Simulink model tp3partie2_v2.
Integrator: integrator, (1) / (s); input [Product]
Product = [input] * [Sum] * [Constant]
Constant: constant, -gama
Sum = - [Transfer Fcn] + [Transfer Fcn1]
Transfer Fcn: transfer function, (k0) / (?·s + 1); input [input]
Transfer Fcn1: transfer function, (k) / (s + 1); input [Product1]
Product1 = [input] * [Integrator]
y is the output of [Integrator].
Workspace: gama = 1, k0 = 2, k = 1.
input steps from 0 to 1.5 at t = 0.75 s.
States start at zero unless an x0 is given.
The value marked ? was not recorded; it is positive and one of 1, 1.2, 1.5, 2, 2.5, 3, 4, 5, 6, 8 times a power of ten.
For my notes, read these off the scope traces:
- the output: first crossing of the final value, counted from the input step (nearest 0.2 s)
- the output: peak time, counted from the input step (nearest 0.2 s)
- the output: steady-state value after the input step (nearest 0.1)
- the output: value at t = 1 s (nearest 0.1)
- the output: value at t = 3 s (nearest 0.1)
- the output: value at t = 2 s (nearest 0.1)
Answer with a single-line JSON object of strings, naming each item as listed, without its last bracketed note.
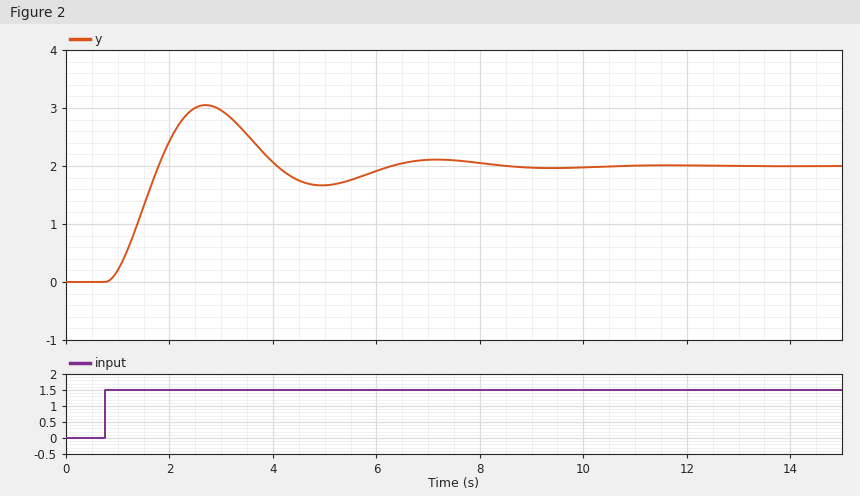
{"the output: first crossing of the final value, counted from the input step": "1.0 s", "the output: peak time, counted from the input step": "2.0 s", "the output: steady-state value after the input step": "2.0", "the output: value at t = 1 s": "0.2", "the output: value at t = 3 s": "3.0", "the output: value at t = 2 s": "2.4"}
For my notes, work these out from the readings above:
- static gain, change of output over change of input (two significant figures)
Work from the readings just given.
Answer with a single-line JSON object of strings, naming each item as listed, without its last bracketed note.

{"static gain, change of output over change of input": "1.3"}
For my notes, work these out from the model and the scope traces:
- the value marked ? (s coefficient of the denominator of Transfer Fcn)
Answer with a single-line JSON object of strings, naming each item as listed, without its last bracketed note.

{"the value marked ?": "0.6"}
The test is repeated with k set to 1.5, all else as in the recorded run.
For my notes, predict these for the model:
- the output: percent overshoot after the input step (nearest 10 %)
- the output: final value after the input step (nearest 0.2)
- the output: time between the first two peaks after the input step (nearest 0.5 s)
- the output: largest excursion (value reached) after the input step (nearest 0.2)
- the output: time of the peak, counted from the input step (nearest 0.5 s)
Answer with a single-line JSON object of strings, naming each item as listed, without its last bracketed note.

{"the output: percent overshoot after the input step": "70 %", "the output: final value after the input step": "1.4", "the output: time between the first two peaks after the input step": "3.5 s", "the output: largest excursion (value reached) after the input step": "2.2", "the output: time of the peak, counted from the input step": "1.5 s"}
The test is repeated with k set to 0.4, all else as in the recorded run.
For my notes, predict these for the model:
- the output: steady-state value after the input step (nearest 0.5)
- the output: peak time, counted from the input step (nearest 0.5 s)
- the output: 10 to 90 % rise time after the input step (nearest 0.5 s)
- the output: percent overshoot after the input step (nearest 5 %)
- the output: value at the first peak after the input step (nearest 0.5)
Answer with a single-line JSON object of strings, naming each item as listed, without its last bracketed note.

{"the output: steady-state value after the input step": "5.0", "the output: peak time, counted from the input step": "3.5 s", "the output: 10 to 90 % rise time after the input step": "1.5 s", "the output: percent overshoot after the input step": "20 %", "the output: value at the first peak after the input step": "6.0"}
